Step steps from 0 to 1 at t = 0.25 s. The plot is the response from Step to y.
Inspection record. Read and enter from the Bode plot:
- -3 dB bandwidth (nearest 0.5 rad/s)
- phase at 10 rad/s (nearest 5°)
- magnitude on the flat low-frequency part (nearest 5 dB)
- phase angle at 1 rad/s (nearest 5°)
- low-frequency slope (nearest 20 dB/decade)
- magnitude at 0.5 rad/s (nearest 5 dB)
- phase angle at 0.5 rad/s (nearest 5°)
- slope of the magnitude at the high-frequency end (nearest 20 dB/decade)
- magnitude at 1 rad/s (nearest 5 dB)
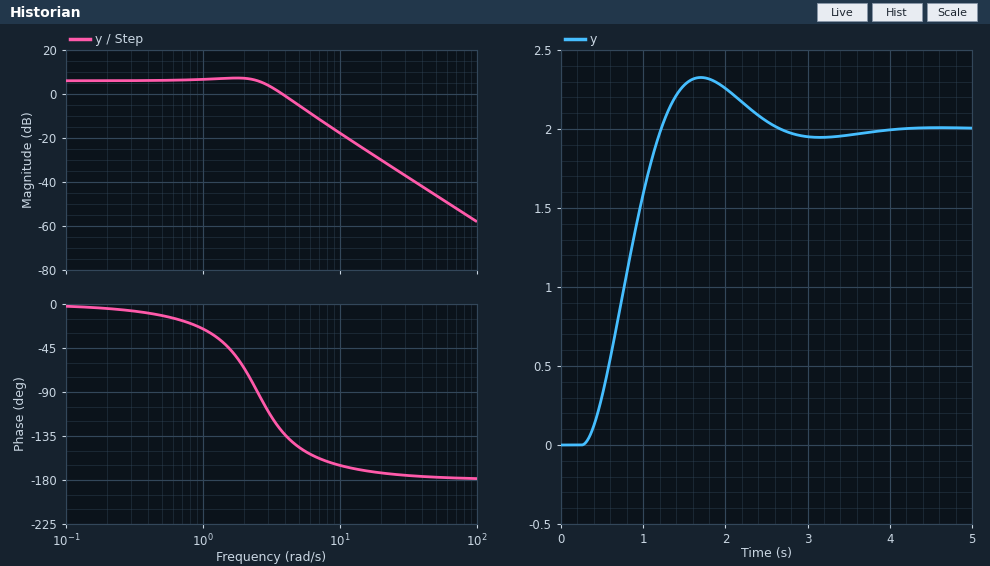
3.0 rad/s
-165°
5 dB
-25°
0 dB/decade
5 dB
-10°
-40 dB/decade
5 dB
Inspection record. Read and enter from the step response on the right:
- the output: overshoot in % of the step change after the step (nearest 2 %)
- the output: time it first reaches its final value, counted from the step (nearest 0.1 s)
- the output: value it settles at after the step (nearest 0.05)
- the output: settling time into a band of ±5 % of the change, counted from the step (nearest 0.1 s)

16 %
1.0 s
2.00
2.1 s
